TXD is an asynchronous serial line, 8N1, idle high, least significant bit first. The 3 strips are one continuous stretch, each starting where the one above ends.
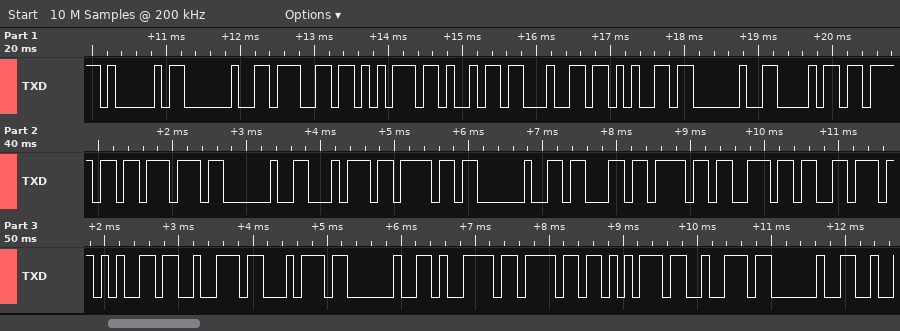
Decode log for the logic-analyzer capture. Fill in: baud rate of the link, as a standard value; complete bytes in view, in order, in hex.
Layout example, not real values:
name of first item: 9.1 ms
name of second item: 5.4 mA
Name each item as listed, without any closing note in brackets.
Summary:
baud rate of the link, as a standard value: 9600 baud
complete bytes in view, in order, in hex: 41 20 67 75 69 64 65 20 68 6F 77 20 74 6F 20 63 6F 6E 76 65 72 74 20 79 6F 75 72 20
